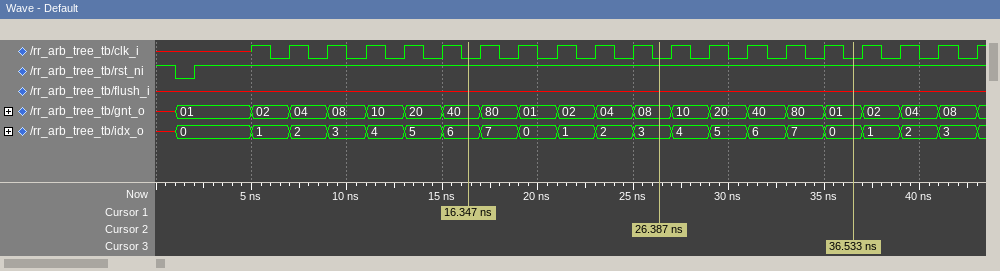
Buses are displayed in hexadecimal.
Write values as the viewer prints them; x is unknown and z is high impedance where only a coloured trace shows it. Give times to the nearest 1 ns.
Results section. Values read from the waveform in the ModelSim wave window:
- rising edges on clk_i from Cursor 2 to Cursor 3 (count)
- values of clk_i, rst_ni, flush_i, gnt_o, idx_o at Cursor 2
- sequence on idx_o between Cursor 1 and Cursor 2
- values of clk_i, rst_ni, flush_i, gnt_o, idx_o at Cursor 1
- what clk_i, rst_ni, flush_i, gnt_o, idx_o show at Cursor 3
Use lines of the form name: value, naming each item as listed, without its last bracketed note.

rising edges on clk_i from Cursor 2 to Cursor 3: 5
values of clk_i, rst_ni, flush_i, gnt_o, idx_o at Cursor 2: clk_i=0, rst_ni=1, flush_i=x, gnt_o=08, idx_o=3
sequence on idx_o between Cursor 1 and Cursor 2: 6, 7, 0, 1, 2, 3
values of clk_i, rst_ni, flush_i, gnt_o, idx_o at Cursor 1: clk_i=0, rst_ni=1, flush_i=x, gnt_o=40, idx_o=6
what clk_i, rst_ni, flush_i, gnt_o, idx_o show at Cursor 3: clk_i=0, rst_ni=1, flush_i=x, gnt_o=01, idx_o=0
